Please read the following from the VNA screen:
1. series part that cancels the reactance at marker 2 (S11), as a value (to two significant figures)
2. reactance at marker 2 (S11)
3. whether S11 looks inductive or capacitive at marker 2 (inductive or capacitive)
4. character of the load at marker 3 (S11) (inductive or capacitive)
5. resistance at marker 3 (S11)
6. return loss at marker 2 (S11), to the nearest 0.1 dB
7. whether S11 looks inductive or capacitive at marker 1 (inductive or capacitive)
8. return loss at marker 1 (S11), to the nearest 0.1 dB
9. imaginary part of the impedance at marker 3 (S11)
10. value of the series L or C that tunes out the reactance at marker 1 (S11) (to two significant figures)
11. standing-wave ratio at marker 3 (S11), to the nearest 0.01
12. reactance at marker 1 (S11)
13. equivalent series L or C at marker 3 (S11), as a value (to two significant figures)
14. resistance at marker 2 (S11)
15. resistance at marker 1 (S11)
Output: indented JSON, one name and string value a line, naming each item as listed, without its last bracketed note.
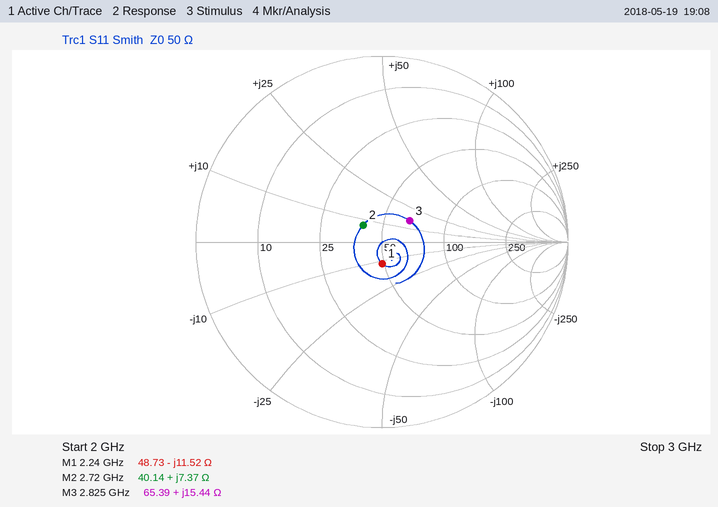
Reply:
{
  "series part that cancels the reactance at marker 2 (S11), as a value": "7.9 pF",
  "reactance at marker 2": "+7.37 Ω",
  "whether S11 looks inductive or capacitive at marker 2": "inductive",
  "character of the load at marker 3 (S11)": "inductive",
  "resistance at marker 3": "65.39 Ω",
  "return loss at marker 2 (S11), to the nearest 0.1 dB": "17.3 dB",
  "whether S11 looks inductive or capacitive at marker 1": "capacitive",
  "return loss at marker 1 (S11), to the nearest 0.1 dB": "18.7 dB",
  "imaginary part of the impedance at marker 3": "+15.44 Ω",
  "value of the series L or C that tunes out the reactance at marker 1 (S11)": "820 pH",
  "standing-wave ratio at marker 3 (S11), to the nearest 0.01": "1.46",
  "reactance at marker 1": "-11.52 Ω",
  "equivalent series L or C at marker 3 (S11), as a value": "870 pH",
  "resistance at marker 2": "40.14 Ω",
  "resistance at marker 1": "48.73 Ω"
}
